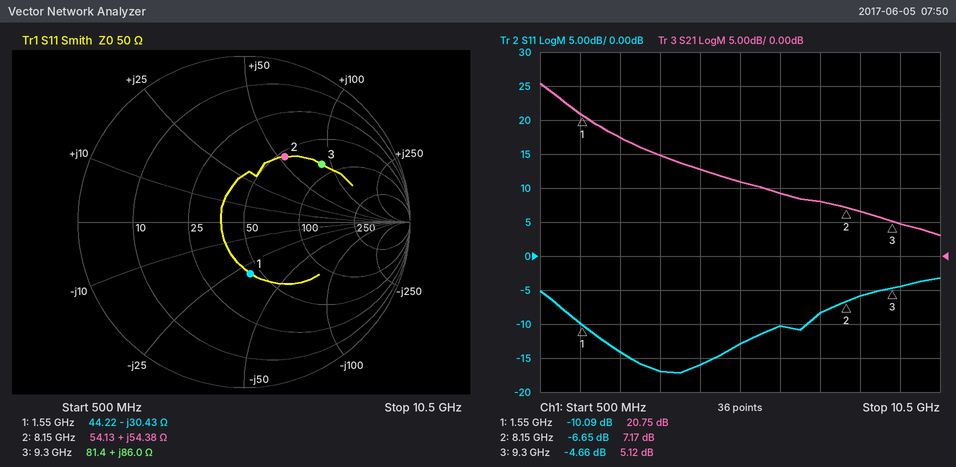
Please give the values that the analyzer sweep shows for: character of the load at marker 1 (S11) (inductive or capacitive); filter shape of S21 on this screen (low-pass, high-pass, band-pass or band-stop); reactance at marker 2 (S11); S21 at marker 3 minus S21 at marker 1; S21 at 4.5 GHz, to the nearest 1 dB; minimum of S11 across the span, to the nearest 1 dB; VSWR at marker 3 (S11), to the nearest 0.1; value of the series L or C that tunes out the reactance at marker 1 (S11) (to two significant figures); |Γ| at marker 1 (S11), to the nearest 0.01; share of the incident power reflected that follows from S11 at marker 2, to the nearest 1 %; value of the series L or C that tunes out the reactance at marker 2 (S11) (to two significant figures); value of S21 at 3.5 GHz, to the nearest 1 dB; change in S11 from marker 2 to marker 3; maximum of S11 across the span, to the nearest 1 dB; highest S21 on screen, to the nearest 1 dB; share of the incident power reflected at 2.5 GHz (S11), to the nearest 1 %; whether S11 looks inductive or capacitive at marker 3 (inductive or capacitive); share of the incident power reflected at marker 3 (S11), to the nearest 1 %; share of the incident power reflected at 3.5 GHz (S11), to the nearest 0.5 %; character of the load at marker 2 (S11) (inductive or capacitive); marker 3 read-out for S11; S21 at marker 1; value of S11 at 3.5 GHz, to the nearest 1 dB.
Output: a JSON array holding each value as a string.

["capacitive", "low-pass", "+54.38 Ω", "-15.63 dB", "13 dB", "-17 dB", "3.8", "3.1 nH", "0.31", "22 %", "360 fF", "15 dB", "1.99 dB", "-3 dB", "25 dB", "4 %", "inductive", "34 %", "2.0 %", "inductive", "-4.66 dB", "20.75 dB", "-17 dB"]
